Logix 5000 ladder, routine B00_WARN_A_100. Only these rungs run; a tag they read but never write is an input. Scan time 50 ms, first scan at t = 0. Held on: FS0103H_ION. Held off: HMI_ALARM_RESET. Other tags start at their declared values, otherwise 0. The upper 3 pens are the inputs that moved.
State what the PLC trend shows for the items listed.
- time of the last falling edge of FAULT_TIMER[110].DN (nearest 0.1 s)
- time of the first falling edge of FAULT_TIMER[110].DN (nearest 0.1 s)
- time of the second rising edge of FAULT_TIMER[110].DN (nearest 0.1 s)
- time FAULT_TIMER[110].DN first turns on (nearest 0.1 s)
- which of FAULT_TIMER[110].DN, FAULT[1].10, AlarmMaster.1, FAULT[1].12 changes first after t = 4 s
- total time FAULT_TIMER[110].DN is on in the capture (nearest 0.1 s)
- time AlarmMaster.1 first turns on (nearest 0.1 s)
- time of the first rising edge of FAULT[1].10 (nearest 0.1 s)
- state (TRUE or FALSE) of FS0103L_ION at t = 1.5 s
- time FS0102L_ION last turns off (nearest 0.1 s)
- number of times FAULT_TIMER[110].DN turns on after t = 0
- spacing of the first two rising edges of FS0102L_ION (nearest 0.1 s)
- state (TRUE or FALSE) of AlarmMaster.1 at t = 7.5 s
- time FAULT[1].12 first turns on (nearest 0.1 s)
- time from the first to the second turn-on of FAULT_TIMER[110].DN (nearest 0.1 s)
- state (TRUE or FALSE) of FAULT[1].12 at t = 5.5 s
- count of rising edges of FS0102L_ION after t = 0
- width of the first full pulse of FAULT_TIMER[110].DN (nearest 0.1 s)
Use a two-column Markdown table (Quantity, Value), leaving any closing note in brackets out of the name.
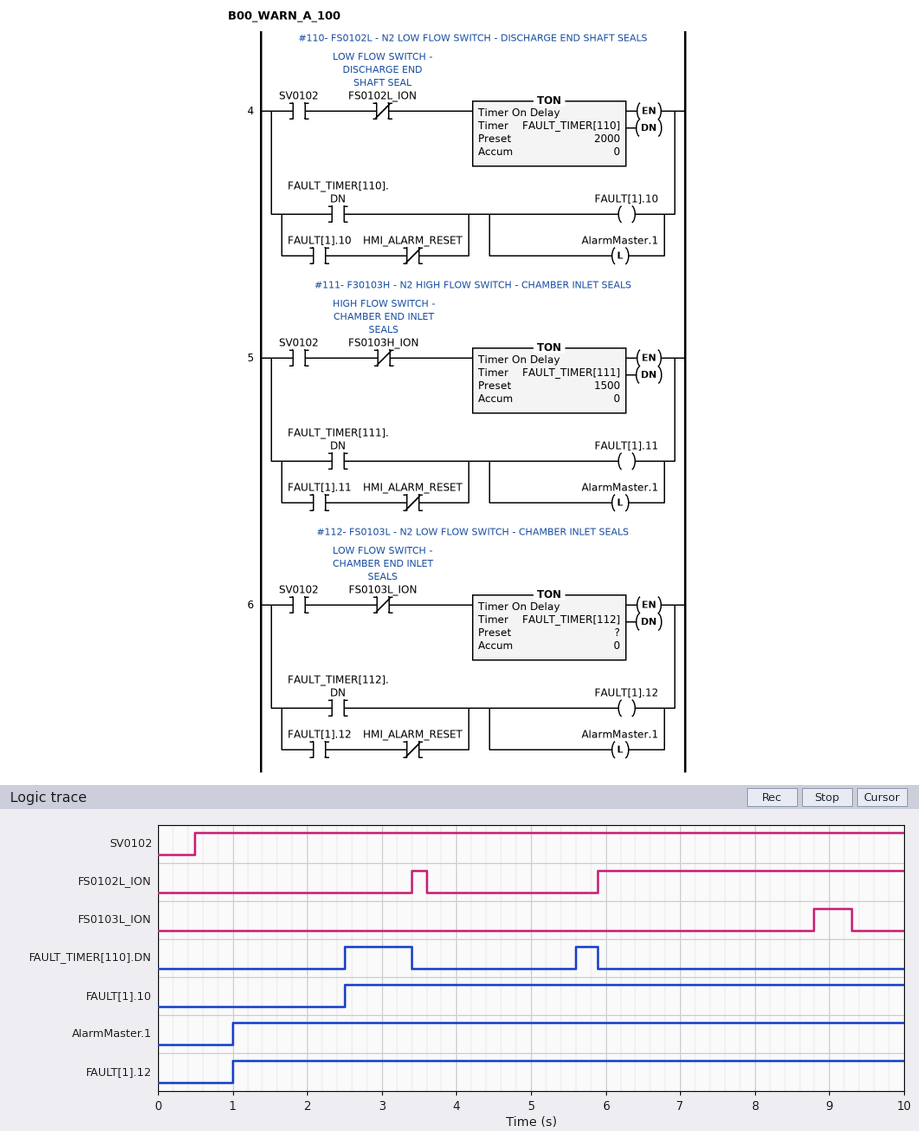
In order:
| Quantity | Value |
|---|---|
| time of the last falling edge of FAULT_TIMER[110].DN | 5.9 s |
| time of the first falling edge of FAULT_TIMER[110].DN | 3.4 s |
| time of the second rising edge of FAULT_TIMER[110].DN | 5.6 s |
| time FAULT_TIMER[110].DN first turns on | 2.5 s |
| which of FAULT_TIMER[110].DN, FAULT[1].10, AlarmMaster.1, FAULT[1].12 changes first after t = 4 s | FAULT_TIMER[110].DN |
| total time FAULT_TIMER[110].DN is on in the capture | 1.2 s |
| time AlarmMaster.1 first turns on | 1.0 s |
| time of the first rising edge of FAULT[1].10 | 2.5 s |
| state (TRUE or FALSE) of FS0103L_ION at t = 1.5 s | FALSE |
| time FS0102L_ION last turns off | 3.6 s |
| number of times FAULT_TIMER[110].DN turns on after t = 0 | 2 |
| spacing of the first two rising edges of FS0102L_ION | 2.5 s |
| state (TRUE or FALSE) of AlarmMaster.1 at t = 7.5 s | TRUE |
| time FAULT[1].12 first turns on | 1.0 s |
| time from the first to the second turn-on of FAULT_TIMER[110].DN | 3.1 s |
| state (TRUE or FALSE) of FAULT[1].12 at t = 5.5 s | TRUE |
| count of rising edges of FS0102L_ION after t = 0 | 2 |
| width of the first full pulse of FAULT_TIMER[110].DN | 0.9 s |
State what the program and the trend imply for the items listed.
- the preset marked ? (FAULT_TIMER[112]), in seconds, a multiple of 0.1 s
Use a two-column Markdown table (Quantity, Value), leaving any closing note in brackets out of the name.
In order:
| Quantity | Value |
|---|---|
| the preset marked ? (FAULT_TIMER[112]), in seconds, a multiple of 0.1 s | 0.5 s |
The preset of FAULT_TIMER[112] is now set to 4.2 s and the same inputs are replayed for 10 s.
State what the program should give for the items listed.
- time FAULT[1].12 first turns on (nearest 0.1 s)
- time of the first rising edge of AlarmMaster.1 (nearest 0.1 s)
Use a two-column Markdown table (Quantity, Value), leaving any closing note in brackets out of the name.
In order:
| Quantity | Value |
|---|---|
| time FAULT[1].12 first turns on | 4.7 s |
| time of the first rising edge of AlarmMaster.1 | 2.5 s |
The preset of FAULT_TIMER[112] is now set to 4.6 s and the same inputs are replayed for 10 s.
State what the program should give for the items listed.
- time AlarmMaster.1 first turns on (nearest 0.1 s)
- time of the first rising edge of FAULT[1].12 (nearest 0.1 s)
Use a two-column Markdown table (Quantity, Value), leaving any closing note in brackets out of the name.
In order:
| Quantity | Value |
|---|---|
| time AlarmMaster.1 first turns on | 2.5 s |
| time of the first rising edge of FAULT[1].12 | 5.1 s |
